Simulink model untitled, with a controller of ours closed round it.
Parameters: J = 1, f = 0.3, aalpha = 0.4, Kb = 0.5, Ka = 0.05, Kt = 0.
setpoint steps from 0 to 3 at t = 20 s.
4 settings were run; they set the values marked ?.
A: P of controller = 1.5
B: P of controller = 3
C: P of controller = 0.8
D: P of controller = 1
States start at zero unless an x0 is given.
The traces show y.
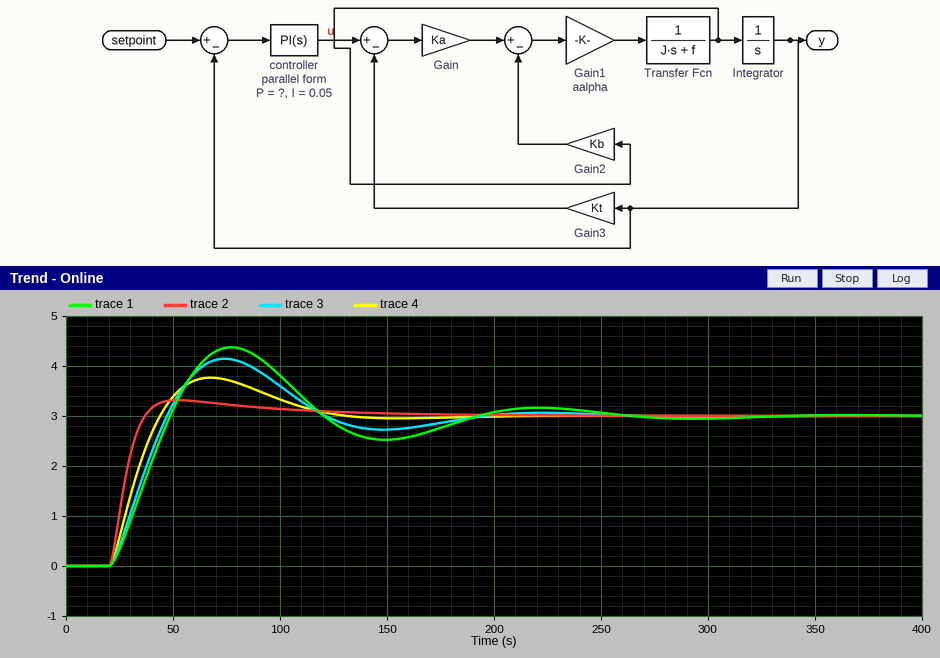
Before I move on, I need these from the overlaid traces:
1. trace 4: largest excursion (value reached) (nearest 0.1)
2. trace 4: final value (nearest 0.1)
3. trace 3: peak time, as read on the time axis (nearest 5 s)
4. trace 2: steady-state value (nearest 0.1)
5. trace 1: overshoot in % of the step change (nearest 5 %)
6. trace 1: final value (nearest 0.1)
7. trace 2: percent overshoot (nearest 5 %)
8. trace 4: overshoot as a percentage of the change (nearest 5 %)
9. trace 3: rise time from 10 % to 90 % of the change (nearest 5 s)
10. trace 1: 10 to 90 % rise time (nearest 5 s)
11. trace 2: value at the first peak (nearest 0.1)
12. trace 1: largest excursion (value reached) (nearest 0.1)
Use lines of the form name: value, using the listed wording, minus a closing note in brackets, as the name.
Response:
trace 4: largest excursion (value reached): 3.8
trace 4: final value: 3.0
trace 3: peak time, as read on the time axis: 75 s
trace 2: steady-state value: 3.0
trace 1: overshoot in % of the step change: 45 %
trace 1: final value: 3.0
trace 2: percent overshoot: 10 %
trace 4: overshoot as a percentage of the change: 25 %
trace 3: rise time from 10 % to 90 % of the change: 20 s
trace 1: 10 to 90 % rise time: 20 s
trace 2: value at the first peak: 3.3
trace 1: largest excursion (value reached): 4.4
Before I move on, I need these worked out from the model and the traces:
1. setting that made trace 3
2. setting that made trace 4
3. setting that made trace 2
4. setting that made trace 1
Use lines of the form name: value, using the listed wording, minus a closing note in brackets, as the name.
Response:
setting that made trace 3: D
setting that made trace 4: A
setting that made trace 2: B
setting that made trace 1: C
